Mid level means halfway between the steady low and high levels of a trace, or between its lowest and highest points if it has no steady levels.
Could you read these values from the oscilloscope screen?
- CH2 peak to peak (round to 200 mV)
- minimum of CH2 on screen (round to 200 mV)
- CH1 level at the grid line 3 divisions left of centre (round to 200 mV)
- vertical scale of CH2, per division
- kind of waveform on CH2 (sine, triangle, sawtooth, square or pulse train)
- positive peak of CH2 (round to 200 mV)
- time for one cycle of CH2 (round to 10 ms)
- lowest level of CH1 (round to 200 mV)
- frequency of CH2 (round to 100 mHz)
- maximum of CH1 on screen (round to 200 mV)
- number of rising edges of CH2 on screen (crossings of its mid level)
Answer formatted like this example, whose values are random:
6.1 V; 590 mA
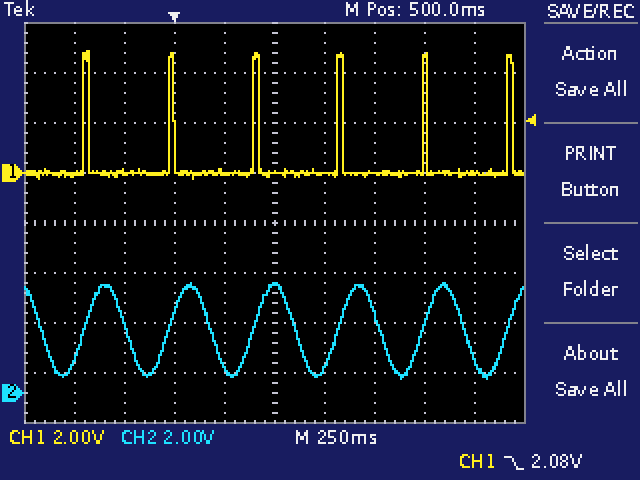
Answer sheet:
3.8 V; 600 mV; 0.0 V; 2 V; sine; 4.4 V; 420 ms; -200 mV; 2.4 Hz; 4.8 V; 6
